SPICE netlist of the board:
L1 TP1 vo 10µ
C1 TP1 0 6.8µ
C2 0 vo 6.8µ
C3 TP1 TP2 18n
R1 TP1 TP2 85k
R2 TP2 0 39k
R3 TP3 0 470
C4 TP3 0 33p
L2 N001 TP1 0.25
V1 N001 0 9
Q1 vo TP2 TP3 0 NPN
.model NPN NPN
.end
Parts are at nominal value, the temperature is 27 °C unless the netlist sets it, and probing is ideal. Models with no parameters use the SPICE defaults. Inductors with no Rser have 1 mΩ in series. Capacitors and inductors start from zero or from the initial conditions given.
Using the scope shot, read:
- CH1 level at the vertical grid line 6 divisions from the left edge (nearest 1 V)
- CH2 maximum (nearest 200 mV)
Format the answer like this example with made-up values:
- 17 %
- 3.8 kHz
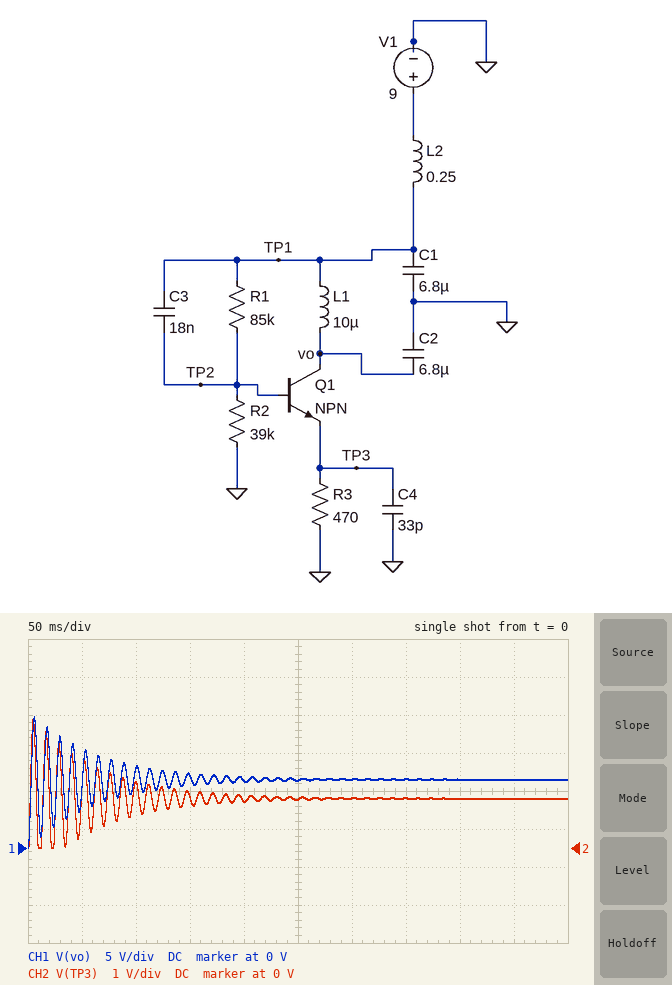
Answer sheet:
- 9 V
- 3.4 V
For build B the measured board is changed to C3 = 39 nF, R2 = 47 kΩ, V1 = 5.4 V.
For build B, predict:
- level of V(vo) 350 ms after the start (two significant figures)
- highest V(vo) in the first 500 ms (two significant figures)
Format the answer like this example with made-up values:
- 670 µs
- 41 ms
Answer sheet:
- 5.4 V
- 10 V
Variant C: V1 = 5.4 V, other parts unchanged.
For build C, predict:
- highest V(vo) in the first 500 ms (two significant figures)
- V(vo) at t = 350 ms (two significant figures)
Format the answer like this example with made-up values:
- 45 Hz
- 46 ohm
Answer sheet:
- 10 V
- 5.4 V
